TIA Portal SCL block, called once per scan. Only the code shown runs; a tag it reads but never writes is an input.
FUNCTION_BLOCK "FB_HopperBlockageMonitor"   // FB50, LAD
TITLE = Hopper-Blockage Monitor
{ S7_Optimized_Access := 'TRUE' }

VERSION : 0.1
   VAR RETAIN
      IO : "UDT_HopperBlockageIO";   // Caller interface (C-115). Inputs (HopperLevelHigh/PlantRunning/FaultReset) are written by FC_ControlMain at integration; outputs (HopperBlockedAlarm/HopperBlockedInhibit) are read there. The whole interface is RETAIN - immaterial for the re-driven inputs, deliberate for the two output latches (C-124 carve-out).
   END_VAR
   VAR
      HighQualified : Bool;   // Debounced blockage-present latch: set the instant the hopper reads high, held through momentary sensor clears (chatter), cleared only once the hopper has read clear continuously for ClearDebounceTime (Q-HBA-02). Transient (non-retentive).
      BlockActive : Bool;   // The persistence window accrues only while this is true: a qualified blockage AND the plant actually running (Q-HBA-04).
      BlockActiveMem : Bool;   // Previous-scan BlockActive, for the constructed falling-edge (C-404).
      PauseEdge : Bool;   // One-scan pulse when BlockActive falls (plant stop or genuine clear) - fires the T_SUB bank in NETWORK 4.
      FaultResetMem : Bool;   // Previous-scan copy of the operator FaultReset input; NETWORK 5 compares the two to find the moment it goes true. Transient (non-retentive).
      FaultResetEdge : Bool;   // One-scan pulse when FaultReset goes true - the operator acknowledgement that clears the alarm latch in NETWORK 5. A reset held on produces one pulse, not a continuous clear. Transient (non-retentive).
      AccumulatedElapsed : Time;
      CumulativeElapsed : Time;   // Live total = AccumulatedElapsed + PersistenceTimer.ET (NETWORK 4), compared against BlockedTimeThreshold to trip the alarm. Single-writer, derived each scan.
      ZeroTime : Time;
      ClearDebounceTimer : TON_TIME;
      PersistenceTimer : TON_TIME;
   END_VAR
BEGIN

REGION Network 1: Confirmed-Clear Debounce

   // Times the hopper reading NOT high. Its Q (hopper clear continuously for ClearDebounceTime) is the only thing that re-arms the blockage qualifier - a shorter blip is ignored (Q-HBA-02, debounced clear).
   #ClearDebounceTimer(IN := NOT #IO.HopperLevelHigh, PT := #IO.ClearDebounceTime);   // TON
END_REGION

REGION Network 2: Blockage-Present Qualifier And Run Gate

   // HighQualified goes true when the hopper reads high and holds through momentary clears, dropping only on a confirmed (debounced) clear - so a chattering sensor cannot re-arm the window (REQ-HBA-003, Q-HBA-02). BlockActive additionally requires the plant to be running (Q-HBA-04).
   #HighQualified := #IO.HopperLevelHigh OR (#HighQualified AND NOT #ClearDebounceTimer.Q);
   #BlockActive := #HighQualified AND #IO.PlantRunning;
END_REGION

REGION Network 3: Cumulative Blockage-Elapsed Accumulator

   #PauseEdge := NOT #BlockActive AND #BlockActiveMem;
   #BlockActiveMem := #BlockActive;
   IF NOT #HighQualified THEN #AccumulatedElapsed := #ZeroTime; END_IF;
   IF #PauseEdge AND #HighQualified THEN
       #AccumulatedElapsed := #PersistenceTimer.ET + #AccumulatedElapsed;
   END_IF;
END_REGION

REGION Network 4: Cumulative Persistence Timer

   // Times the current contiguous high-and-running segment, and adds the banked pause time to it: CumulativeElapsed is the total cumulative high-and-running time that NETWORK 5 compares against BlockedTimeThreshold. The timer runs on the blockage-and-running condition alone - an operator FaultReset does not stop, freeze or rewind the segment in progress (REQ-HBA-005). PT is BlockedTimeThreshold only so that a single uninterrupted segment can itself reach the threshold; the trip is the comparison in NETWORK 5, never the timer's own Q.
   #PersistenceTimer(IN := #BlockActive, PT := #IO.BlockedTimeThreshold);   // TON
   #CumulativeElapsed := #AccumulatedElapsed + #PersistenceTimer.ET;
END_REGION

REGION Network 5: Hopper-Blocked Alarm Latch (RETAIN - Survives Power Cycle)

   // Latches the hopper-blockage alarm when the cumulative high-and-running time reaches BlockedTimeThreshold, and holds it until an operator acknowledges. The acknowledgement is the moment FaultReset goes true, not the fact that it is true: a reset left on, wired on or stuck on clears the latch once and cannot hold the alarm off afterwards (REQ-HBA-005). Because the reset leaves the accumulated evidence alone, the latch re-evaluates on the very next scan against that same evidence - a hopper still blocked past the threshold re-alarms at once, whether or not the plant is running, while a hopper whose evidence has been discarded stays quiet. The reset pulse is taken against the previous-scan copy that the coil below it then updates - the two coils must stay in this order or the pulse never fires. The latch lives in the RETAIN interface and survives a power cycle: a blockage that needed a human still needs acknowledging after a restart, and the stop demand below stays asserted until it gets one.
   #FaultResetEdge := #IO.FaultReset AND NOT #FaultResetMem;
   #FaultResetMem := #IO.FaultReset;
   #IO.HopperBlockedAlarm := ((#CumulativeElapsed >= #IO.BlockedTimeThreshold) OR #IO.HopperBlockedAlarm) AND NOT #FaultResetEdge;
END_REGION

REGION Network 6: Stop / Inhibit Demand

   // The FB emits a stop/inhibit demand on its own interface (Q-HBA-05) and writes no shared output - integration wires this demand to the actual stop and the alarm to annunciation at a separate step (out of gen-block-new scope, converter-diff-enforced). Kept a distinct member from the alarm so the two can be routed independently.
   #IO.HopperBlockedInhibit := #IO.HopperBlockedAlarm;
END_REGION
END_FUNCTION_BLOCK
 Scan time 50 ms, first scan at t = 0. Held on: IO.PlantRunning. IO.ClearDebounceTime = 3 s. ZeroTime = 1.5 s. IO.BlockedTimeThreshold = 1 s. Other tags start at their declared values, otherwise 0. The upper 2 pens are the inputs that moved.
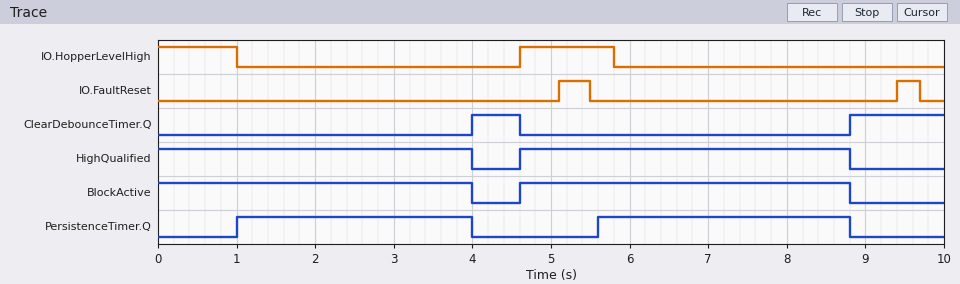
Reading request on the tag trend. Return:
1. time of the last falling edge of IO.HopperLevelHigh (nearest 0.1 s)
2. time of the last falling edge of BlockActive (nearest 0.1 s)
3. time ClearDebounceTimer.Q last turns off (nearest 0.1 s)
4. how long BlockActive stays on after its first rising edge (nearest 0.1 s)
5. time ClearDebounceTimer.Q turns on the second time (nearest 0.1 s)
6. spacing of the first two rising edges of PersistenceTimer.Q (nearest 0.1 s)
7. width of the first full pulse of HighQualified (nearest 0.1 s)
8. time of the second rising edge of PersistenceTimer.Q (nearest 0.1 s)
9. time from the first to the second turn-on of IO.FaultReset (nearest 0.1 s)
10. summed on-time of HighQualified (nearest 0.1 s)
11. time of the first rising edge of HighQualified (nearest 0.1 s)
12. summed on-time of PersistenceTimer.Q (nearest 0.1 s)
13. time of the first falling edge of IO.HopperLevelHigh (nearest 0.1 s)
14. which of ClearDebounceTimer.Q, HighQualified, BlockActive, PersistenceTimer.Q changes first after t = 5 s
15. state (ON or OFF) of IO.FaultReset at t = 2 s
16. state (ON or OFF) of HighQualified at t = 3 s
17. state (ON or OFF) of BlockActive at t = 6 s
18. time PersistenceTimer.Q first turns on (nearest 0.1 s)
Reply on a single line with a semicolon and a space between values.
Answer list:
5.8 s; 8.8 s; 4.6 s; 4.2 s; 8.8 s; 4.6 s; 4.2 s; 5.6 s; 4.3 s; 8.2 s; 4.6 s; 6.2 s; 1.0 s; PersistenceTimer.Q; OFF; ON; ON; 1.0 s
